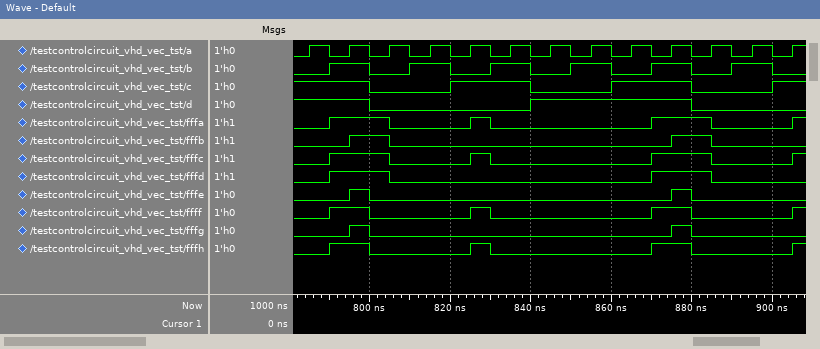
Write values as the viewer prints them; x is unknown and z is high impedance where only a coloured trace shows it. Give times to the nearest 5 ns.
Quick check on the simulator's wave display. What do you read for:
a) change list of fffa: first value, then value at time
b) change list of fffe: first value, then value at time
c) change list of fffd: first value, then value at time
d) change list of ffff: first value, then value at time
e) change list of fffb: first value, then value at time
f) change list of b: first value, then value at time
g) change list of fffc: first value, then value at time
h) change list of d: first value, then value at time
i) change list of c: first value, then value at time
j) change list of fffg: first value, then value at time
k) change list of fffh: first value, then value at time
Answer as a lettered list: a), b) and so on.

a) 0, 1 at 790 ns, 0 at 805 ns, 1 at 825 ns, 0 at 830 ns, 1 at 870 ns, 0 at 885 ns, 1 at 905 ns
b) 0, 1 at 795 ns, 0 at 800 ns, 1 at 875 ns, 0 at 880 ns
c) 0, 1 at 790 ns, 0 at 805 ns, 1 at 870 ns, 0 at 885 ns
d) 0, 1 at 790 ns, 0 at 800 ns, 1 at 825 ns, 0 at 830 ns, 1 at 870 ns, 0 at 880 ns, 1 at 905 ns
e) 0, 1 at 795 ns, 0 at 805 ns, 1 at 875 ns, 0 at 885 ns
f) 0, 1 at 790 ns, 0 at 800 ns, 1 at 810 ns, 0 at 820 ns, 1 at 830 ns, 0 at 840 ns, 1 at 850 ns, 0 at 860 ns, 1 at 870 ns, 0 at 880 ns, 1 at 890 ns, 0 at 900 ns
g) 0, 1 at 790 ns, 0 at 805 ns, 1 at 825 ns, 0 at 830 ns, 1 at 870 ns, 0 at 885 ns, 1 at 905 ns
h) 1, 0 at 800 ns, 1 at 840 ns, 0 at 880 ns
i) 1, 0 at 800 ns, 1 at 820 ns, 0 at 840 ns, 1 at 860 ns, 0 at 880 ns, 1 at 900 ns
j) 0, 1 at 795 ns, 0 at 800 ns, 1 at 875 ns, 0 at 880 ns
k) 0, 1 at 790 ns, 0 at 800 ns, 1 at 825 ns, 0 at 830 ns, 1 at 870 ns, 0 at 880 ns, 1 at 905 ns
